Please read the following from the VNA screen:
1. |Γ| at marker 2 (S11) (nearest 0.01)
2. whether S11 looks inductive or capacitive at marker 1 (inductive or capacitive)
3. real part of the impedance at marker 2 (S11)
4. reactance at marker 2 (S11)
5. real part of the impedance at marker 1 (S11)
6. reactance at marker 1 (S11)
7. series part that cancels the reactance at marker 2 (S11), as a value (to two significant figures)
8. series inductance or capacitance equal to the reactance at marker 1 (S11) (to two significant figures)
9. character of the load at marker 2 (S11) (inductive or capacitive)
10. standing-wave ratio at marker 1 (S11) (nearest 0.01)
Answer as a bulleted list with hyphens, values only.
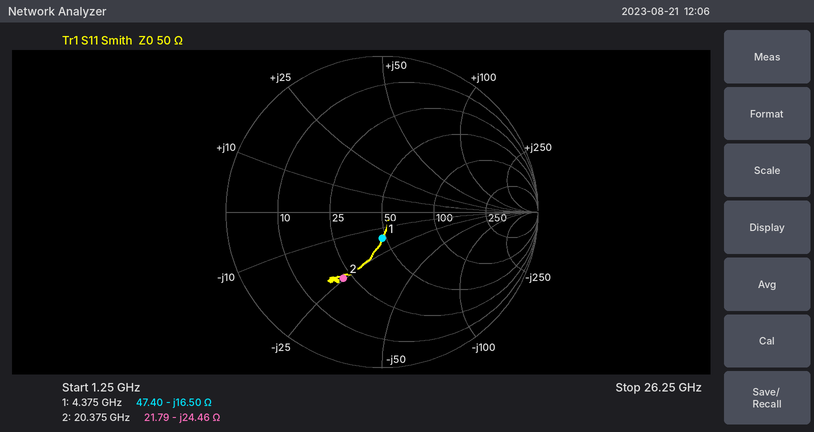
- 0.49
- capacitive
- 21.79 Ω
- -24.46 Ω
- 47.40 Ω
- -16.50 Ω
- 190 pH
- 2.2 pF
- capacitive
- 1.41
